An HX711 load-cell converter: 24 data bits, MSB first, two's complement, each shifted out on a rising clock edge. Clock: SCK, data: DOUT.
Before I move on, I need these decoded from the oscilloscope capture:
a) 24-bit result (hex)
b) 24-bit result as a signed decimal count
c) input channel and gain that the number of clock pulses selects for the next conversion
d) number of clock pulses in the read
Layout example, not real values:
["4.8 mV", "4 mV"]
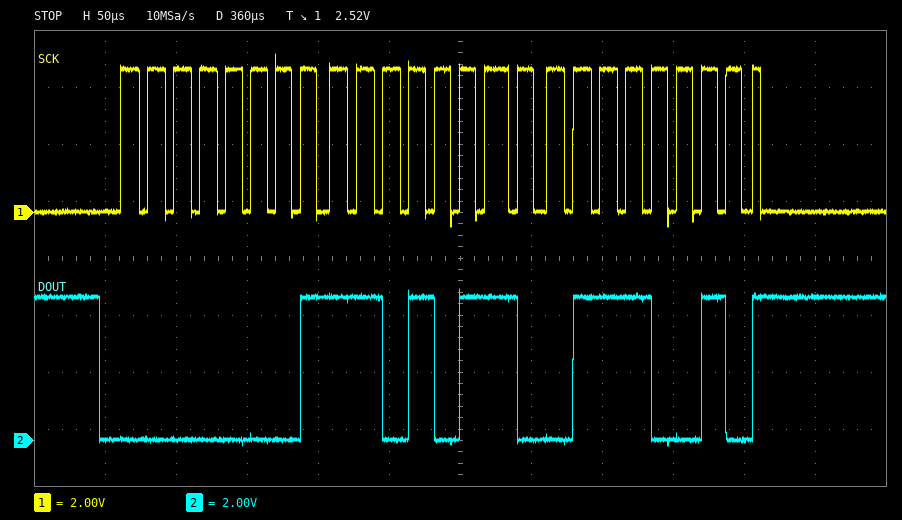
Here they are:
["0x01D672", "120434", "channel A, gain 128", "25"]
